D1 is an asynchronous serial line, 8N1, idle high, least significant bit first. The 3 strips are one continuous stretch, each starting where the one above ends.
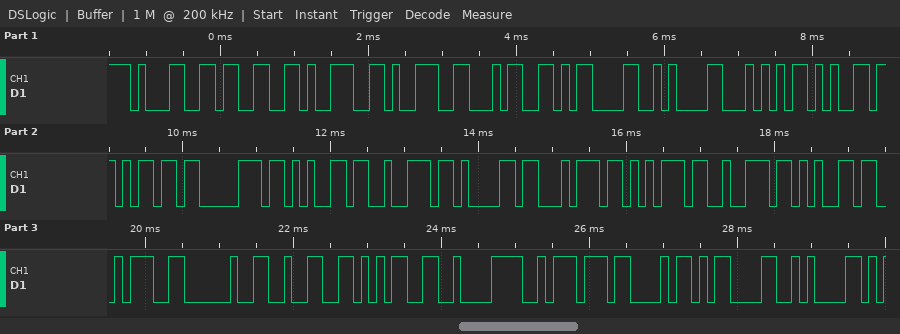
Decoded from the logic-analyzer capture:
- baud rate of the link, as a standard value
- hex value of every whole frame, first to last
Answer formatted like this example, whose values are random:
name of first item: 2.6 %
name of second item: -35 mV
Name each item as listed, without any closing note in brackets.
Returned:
baud rate of the link, as a standard value: 9600 baud
hex value of every whole frame, first to last: 0x31 0x33 0x39 0x39 0x34 0x0D 0x0A 0x54 0x65 0x6D 0x70 0x65 0x72 0x61 0x74 0x75 0x72 0x65 0x3A 0x20 0x32 0x35 0xC2 0xBA 0x43 0x0D 0x0A
